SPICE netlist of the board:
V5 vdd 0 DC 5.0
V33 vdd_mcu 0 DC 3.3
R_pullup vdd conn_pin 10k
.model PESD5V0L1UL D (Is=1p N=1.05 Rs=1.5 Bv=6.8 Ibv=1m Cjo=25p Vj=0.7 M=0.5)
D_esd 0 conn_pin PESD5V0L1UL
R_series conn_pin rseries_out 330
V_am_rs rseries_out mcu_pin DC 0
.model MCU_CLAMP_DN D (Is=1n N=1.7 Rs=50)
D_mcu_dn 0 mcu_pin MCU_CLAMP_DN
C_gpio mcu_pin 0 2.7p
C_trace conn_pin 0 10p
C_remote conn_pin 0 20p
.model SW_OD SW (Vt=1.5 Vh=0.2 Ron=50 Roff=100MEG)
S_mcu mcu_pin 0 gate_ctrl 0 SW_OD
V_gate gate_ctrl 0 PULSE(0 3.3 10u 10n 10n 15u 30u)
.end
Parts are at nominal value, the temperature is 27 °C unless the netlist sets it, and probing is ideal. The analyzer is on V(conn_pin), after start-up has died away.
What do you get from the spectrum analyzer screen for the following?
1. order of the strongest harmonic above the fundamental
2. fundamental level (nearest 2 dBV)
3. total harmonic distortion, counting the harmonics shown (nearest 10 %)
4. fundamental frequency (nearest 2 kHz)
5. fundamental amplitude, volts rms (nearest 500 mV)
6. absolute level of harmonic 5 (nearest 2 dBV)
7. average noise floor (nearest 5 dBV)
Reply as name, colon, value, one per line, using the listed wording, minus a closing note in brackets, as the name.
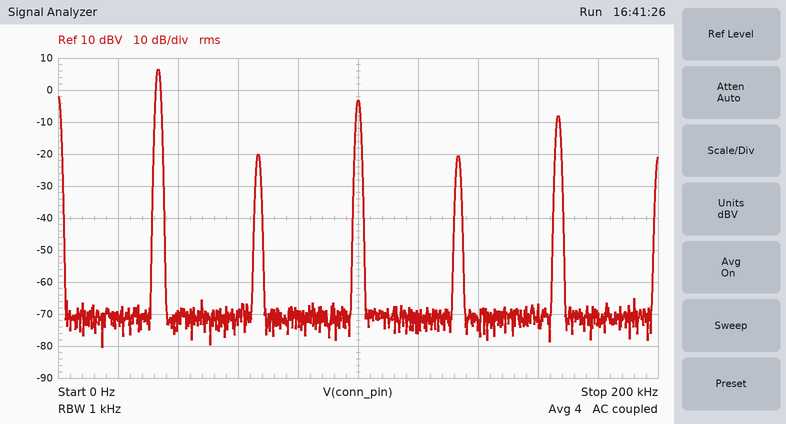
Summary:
order of the strongest harmonic above the fundamental: 3
fundamental level: 6 dBV
total harmonic distortion, counting the harmonics shown: 40 %
fundamental frequency: 34 kHz
fundamental amplitude, volts rms: 2.0 V
absolute level of harmonic 5: -8 dBV
average noise floor: -70 dBV
